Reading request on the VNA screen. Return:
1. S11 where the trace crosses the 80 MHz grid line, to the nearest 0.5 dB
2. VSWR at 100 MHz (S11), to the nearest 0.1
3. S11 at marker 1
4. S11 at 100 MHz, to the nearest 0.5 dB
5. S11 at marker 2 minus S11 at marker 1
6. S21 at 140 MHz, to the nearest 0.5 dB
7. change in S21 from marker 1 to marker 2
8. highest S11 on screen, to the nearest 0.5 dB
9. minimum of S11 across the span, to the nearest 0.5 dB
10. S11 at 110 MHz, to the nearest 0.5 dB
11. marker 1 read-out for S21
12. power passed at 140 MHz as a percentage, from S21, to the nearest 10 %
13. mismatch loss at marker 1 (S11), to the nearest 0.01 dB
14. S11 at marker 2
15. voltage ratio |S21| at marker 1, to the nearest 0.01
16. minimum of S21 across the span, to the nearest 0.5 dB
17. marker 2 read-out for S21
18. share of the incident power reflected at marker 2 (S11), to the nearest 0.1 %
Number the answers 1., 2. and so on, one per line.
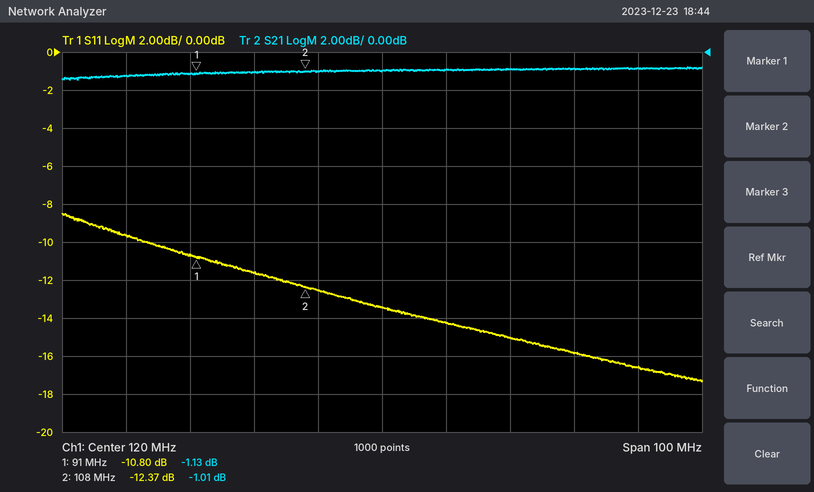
1. -9.5 dB
2. 1.7
3. -10.80 dB
4. -11.5 dB
5. -1.57 dB
6. -1.0 dB
7. 0.12 dB
8. -8.5 dB
9. -17.5 dB
10. -12.5 dB
11. -1.13 dB
12. 80 %
13. 0.38 dB
14. -12.37 dB
15. 0.88
16. -1.5 dB
17. -1.01 dB
18. 5.8 %
